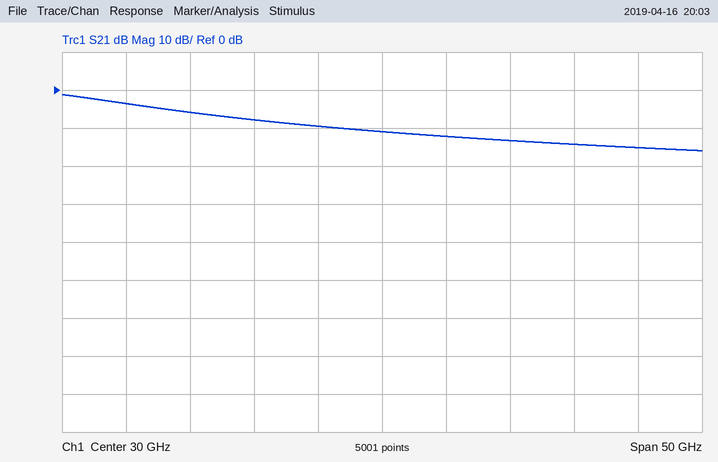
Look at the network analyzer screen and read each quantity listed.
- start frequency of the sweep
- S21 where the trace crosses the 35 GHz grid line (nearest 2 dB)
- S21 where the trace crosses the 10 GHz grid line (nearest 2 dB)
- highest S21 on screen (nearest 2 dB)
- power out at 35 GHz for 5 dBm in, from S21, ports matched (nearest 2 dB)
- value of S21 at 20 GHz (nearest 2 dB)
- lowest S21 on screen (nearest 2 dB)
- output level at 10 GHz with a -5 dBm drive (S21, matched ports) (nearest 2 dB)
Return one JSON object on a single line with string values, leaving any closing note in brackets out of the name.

{"start frequency of the sweep": "5 GHz", "S21 where the trace crosses the 35 GHz grid line": "-12 dB", "S21 where the trace crosses the 10 GHz grid line": "-4 dB", "highest S21 on screen": "-2 dB", "power out at 35 GHz for 5 dBm in, from S21, ports matched": "-8 dBm", "value of S21 at 20 GHz": "-8 dB", "lowest S21 on screen": "-16 dB", "output level at 10 GHz with a -5 dBm drive (S21, matched ports)": "-8 dBm"}
